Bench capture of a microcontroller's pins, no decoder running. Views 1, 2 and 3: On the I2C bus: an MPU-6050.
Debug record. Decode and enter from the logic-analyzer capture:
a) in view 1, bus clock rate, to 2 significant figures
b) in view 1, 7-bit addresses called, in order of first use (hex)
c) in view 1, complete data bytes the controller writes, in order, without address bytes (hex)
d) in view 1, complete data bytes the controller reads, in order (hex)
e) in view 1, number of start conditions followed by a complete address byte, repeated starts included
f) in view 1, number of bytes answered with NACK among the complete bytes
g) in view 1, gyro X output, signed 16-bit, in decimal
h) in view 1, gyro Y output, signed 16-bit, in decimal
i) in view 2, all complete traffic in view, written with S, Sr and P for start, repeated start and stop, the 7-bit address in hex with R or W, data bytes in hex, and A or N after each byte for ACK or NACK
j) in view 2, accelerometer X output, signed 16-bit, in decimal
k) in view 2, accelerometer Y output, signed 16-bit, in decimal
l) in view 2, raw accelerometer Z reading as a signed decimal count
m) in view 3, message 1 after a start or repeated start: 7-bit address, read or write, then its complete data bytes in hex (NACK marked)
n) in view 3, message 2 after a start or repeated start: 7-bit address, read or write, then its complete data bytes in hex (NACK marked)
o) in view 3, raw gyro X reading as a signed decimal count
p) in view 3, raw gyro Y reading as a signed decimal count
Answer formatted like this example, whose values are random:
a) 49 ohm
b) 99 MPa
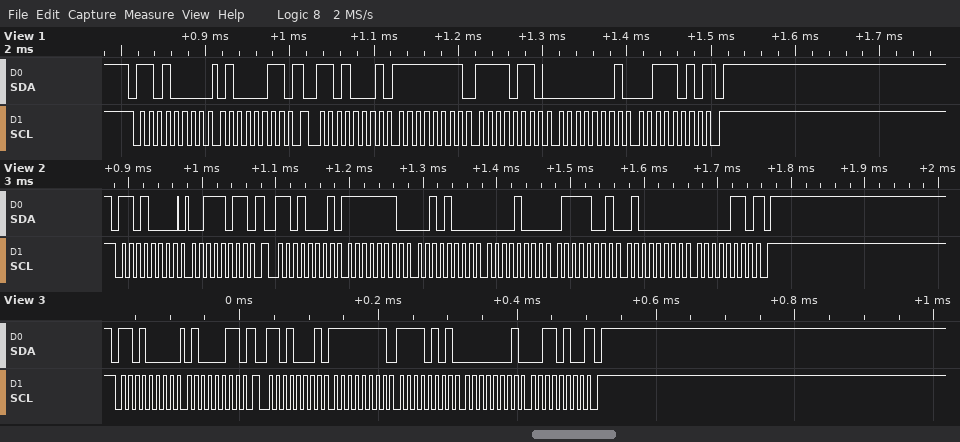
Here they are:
a) 100 kHz
b) 0x68
c) 43
d) FF F6 01 3A
e) 2
f) 1
g) -10
h) 314
i) S 68W A 3B A Sr 68R A FE A 28 A 08 A 79 A 40 A 06 N P
j) -472
k) 2169
l) 16390
m) 0x68 write: 43
n) 0x68 read: FF F5 01 34 NACK
o) -11
p) 308
